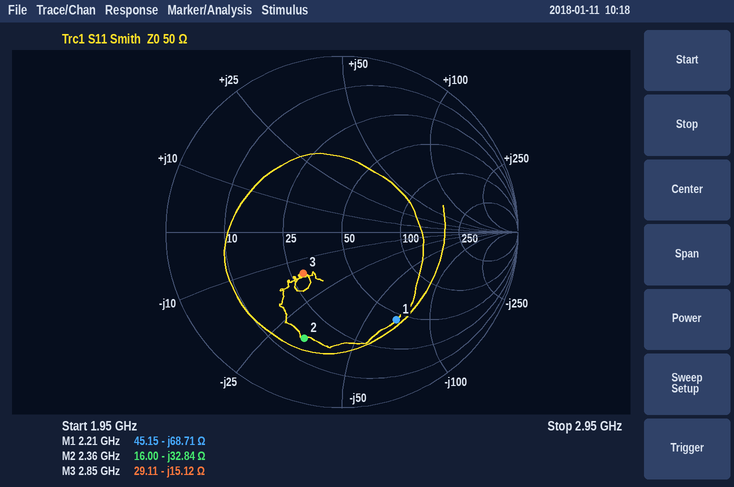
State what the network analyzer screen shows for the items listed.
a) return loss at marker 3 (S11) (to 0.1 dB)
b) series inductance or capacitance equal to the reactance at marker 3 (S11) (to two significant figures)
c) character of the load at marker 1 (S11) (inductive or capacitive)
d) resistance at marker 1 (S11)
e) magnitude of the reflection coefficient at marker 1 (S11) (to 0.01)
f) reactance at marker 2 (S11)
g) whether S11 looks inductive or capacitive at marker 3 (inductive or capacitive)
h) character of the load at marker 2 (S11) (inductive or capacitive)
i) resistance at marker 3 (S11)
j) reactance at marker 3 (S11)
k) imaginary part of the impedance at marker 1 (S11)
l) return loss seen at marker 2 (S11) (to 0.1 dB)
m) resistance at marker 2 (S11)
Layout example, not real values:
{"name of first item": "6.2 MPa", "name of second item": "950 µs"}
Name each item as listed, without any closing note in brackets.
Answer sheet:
{"return loss at marker 3 (S11)": "9.9 dB", "series inductance or capacitance equal to the reactance at marker 3 (S11)": "3.7 pF", "character of the load at marker 1 (S11)": "capacitive", "resistance at marker 1": "45.15 Ω", "magnitude of the reflection coefficient at marker 1 (S11)": "0.59", "reactance at marker 2": "-32.84 Ω", "whether S11 looks inductive or capacitive at marker 3": "capacitive", "character of the load at marker 2 (S11)": "capacitive", "resistance at marker 3": "29.11 Ω", "reactance at marker 3": "-15.12 Ω", "imaginary part of the impedance at marker 1": "-68.71 Ω", "return loss seen at marker 2 (S11)": "3.9 dB", "resistance at marker 2": "16.00 Ω"}
